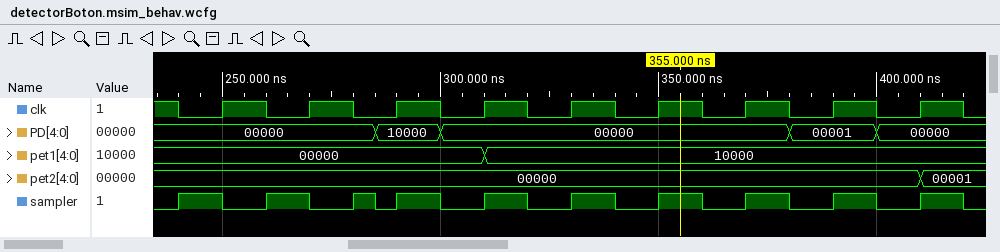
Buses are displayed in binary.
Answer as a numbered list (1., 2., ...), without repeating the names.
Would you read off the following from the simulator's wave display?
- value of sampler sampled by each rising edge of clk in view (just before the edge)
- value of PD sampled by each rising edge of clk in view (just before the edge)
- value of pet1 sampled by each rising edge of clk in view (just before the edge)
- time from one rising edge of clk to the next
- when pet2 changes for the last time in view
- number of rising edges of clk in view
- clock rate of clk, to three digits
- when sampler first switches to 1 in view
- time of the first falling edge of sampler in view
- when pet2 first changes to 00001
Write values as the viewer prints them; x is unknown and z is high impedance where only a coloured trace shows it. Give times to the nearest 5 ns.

1. 1 1 0 0 0 0 0 0 0
2. 00000, 00000, 10000, 00000, 00000, 00000, 00000, 00001, 00000
3. 00000, 00000, 00000, 00000, 10000, 10000, 10000, 10000, 10000
4. 20 ns
5. 410 ns
6. 9
7. 50.0 MHz
8. 240 ns
9. 250 ns
10. 410 ns
